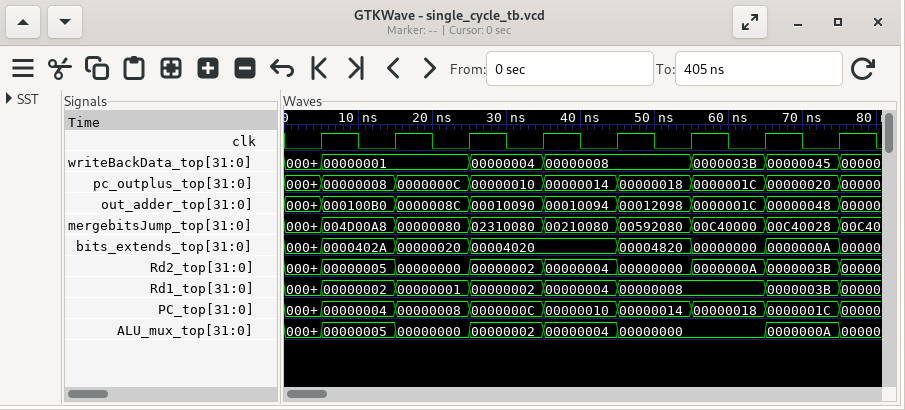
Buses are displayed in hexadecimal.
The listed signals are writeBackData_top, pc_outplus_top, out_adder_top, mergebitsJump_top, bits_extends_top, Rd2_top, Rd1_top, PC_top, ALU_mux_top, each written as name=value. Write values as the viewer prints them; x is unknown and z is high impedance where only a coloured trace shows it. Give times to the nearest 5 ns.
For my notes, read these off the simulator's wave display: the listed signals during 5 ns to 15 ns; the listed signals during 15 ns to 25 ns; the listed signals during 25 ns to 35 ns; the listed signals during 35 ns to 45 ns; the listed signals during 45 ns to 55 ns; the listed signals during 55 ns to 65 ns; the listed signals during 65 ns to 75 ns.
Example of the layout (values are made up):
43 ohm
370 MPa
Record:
writeBackData_top=00000001, pc_outplus_top=00000008, out_adder_top=000100B0, mergebitsJump_top=004D00A8, bits_extends_top=0000402A, Rd2_top=00000005, Rd1_top=00000002, PC_top=00000004, ALU_mux_top=00000005
writeBackData_top=00000001, pc_outplus_top=0000000C, out_adder_top=0000008C, mergebitsJump_top=00000080, bits_extends_top=00000020, Rd2_top=00000000, Rd1_top=00000001, PC_top=00000008, ALU_mux_top=00000000
writeBackData_top=00000004, pc_outplus_top=00000010, out_adder_top=00010090, mergebitsJump_top=02310080, bits_extends_top=00004020, Rd2_top=00000002, Rd1_top=00000002, PC_top=0000000C, ALU_mux_top=00000002
writeBackData_top=00000008, pc_outplus_top=00000014, out_adder_top=00010094, mergebitsJump_top=00210080, bits_extends_top=00004020, Rd2_top=00000004, Rd1_top=00000004, PC_top=00000010, ALU_mux_top=00000004
writeBackData_top=00000008, pc_outplus_top=00000018, out_adder_top=00012098, mergebitsJump_top=00592080, bits_extends_top=00004820, Rd2_top=00000000, Rd1_top=00000008, PC_top=00000014, ALU_mux_top=00000000
writeBackData_top=0000003B, pc_outplus_top=0000001C, out_adder_top=0000001C, mergebitsJump_top=00C40000, bits_extends_top=00000000, Rd2_top=0000000A, Rd1_top=00000008, PC_top=00000018, ALU_mux_top=00000000
writeBackData_top=00000045, pc_outplus_top=00000020, out_adder_top=00000048, mergebitsJump_top=00C40028, bits_extends_top=0000000A, Rd2_top=0000003B, Rd1_top=0000003B, PC_top=0000001C, ALU_mux_top=0000000A
